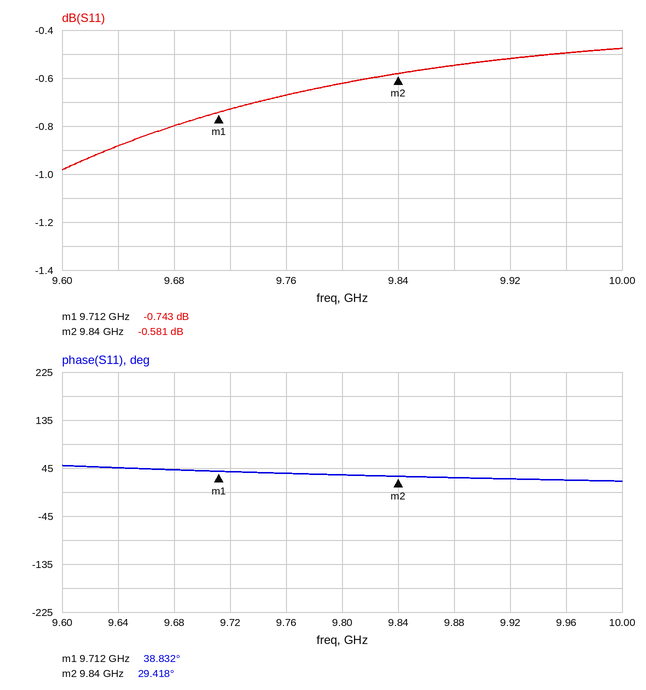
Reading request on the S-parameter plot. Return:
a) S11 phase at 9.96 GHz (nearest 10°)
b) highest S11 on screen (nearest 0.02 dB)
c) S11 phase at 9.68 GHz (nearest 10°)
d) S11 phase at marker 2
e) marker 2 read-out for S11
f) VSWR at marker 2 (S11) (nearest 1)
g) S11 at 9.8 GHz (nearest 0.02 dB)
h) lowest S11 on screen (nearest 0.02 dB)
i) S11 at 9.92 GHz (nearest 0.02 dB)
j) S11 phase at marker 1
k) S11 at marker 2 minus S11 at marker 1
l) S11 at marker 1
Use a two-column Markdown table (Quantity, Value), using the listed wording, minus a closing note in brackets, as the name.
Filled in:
| Quantity | Value |
|---|---|
| S11 phase at 9.96 GHz | 20° |
| highest S11 on screen | -0.48 dB |
| S11 phase at 9.68 GHz | 40° |
| S11 phase at marker 2 | 29.418° |
| marker 2 read-out for S11 | -0.581 dB |
| VSWR at marker 2 (S11) | 30 |
| S11 at 9.8 GHz | -0.62 dB |
| lowest S11 on screen | -0.98 dB |
| S11 at 9.92 GHz | -0.52 dB |
| S11 phase at marker 1 | 38.832° |
| S11 at marker 2 minus S11 at marker 1 | 0.162 dB |
| S11 at marker 1 | -0.743 dB |
